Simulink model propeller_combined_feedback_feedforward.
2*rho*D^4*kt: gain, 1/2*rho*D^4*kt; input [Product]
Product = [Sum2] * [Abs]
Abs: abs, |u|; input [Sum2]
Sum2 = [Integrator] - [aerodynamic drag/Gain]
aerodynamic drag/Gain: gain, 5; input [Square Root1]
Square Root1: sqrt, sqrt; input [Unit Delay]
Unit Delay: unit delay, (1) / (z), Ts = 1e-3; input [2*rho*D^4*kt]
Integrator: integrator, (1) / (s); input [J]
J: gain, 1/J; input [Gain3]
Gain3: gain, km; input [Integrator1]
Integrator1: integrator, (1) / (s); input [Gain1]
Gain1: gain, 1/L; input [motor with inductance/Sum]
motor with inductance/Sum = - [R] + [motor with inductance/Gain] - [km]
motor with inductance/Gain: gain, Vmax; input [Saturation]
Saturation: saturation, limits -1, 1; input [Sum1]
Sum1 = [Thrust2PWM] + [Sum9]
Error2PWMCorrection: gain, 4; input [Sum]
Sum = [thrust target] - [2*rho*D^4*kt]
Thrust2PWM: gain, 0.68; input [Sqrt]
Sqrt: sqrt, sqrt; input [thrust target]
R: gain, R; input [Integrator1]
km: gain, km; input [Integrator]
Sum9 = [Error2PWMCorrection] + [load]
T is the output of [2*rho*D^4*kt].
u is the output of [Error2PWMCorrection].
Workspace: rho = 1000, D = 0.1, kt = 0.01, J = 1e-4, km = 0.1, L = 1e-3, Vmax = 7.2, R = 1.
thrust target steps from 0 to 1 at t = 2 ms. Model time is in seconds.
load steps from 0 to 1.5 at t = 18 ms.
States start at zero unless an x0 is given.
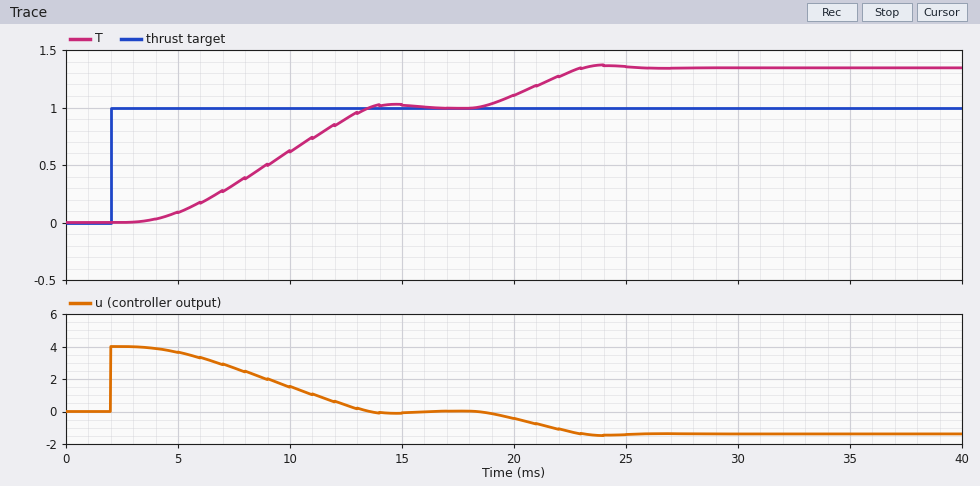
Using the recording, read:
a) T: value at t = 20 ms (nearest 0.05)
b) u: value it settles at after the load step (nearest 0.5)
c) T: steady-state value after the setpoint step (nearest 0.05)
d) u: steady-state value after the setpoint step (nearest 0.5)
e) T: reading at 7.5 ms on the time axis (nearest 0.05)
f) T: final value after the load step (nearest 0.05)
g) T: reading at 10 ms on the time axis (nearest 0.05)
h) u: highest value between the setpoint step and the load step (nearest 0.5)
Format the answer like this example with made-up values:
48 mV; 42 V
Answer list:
1.10; -1.5; 1.00; 0.0; 0.35; 1.35; 0.60; 4.0
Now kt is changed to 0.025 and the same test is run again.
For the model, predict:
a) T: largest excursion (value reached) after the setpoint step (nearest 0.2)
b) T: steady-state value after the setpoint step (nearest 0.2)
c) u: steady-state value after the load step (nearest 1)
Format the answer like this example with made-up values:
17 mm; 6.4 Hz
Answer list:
1.2; 1.0; -2
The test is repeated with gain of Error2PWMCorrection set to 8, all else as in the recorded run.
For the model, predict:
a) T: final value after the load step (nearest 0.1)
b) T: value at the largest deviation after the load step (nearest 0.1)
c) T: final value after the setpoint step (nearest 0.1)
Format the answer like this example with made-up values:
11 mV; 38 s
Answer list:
1.2; 1.2; 1.0
